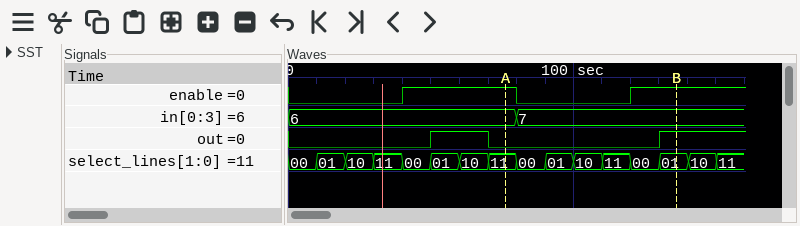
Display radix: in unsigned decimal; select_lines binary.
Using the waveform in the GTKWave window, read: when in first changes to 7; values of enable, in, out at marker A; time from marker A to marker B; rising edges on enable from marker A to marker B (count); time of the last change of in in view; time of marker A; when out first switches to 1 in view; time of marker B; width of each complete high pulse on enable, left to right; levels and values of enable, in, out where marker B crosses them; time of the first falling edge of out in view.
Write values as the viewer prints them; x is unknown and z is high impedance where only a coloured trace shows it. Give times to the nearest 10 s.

80 s
enable=1, in=6, out=0
60 s
1
80 s
80 s
50 s
140 s
40 s
enable=1, in=7, out=1
70 s
